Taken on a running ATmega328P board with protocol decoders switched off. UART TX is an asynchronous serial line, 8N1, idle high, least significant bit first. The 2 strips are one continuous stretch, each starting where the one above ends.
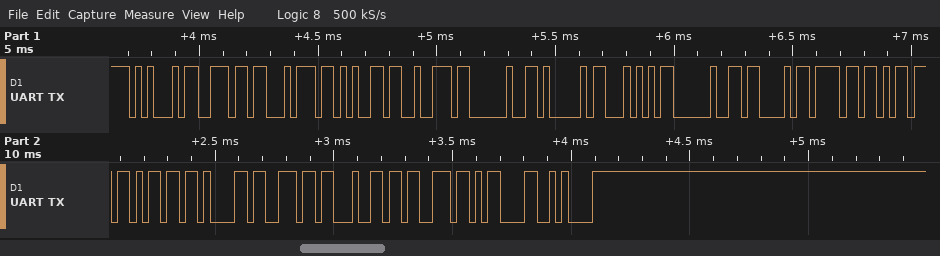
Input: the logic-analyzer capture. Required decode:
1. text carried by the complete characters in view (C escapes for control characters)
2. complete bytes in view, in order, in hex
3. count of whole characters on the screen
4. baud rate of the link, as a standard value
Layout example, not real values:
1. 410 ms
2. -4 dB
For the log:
1. "Enter AT Commands\r\n"
2. 45 6E 74 65 72 20 41 54 20 43 6F 6D 6D 61 6E 64 73 0D 0A
3. 19
4. 38400 baud
